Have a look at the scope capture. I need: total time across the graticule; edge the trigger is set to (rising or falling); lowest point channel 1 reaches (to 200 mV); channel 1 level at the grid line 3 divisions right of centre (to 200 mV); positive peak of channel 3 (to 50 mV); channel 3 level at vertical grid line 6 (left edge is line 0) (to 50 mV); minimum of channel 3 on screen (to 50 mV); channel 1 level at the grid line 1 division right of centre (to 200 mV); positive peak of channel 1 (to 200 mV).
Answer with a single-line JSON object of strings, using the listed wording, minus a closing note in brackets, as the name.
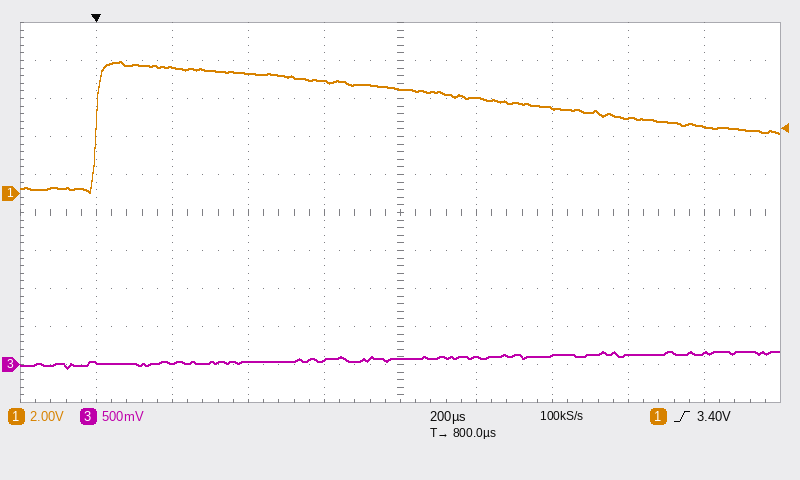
{"total time across the graticule": "2 ms", "edge the trigger is set to": "rising", "lowest point channel 1 reaches": "0.0 V", "channel 1 level at the grid line 3 divisions right of centre": "4.0 V", "positive peak of channel 3": "150 mV", "channel 3 level at vertical grid line 6 (left edge is line 0)": "100 mV", "minimum of channel 3 on screen": "-50 mV", "channel 1 level at the grid line 1 division right of centre": "5.0 V", "positive peak of channel 1": "7.0 V"}
